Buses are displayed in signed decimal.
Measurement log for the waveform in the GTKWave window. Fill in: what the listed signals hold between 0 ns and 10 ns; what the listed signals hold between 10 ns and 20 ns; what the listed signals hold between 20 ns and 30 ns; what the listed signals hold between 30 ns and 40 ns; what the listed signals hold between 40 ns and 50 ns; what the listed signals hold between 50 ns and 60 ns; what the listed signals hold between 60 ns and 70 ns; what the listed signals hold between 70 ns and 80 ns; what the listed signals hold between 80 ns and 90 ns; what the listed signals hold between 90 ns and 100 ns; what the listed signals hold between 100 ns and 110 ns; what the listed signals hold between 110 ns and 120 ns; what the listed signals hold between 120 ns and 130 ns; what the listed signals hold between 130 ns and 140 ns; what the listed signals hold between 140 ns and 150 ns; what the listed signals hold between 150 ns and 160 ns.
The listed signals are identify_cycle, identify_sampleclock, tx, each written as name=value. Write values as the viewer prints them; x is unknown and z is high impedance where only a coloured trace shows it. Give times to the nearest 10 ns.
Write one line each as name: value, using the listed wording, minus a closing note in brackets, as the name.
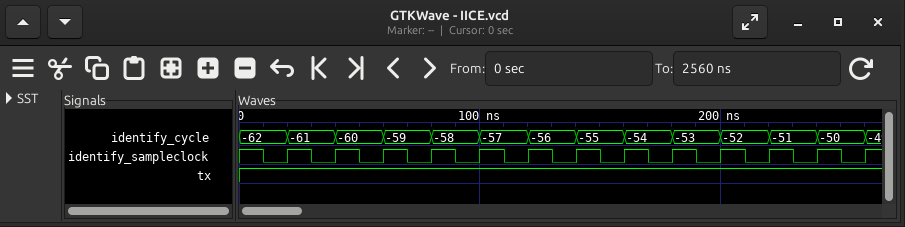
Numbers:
what the listed signals hold between 0 ns and 10 ns: identify_cycle=-62, identify_sampleclock=1, tx=1
what the listed signals hold between 10 ns and 20 ns: identify_cycle=-62, identify_sampleclock=0, tx=1
what the listed signals hold between 20 ns and 30 ns: identify_cycle=-61, identify_sampleclock=1, tx=1
what the listed signals hold between 30 ns and 40 ns: identify_cycle=-61, identify_sampleclock=0, tx=1
what the listed signals hold between 40 ns and 50 ns: identify_cycle=-60, identify_sampleclock=1, tx=1
what the listed signals hold between 50 ns and 60 ns: identify_cycle=-60, identify_sampleclock=0, tx=1
what the listed signals hold between 60 ns and 70 ns: identify_cycle=-59, identify_sampleclock=1, tx=1
what the listed signals hold between 70 ns and 80 ns: identify_cycle=-59, identify_sampleclock=0, tx=1
what the listed signals hold between 80 ns and 90 ns: identify_cycle=-58, identify_sampleclock=1, tx=1
what the listed signals hold between 90 ns and 100 ns: identify_cycle=-58, identify_sampleclock=0, tx=1
what the listed signals hold between 100 ns and 110 ns: identify_cycle=-57, identify_sampleclock=1, tx=1
what the listed signals hold between 110 ns and 120 ns: identify_cycle=-57, identify_sampleclock=0, tx=1
what the listed signals hold between 120 ns and 130 ns: identify_cycle=-56, identify_sampleclock=1, tx=1
what the listed signals hold between 130 ns and 140 ns: identify_cycle=-56, identify_sampleclock=0, tx=1
what the listed signals hold between 140 ns and 150 ns: identify_cycle=-55, identify_sampleclock=1, tx=1
what the listed signals hold between 150 ns and 160 ns: identify_cycle=-55, identify_sampleclock=0, tx=1
